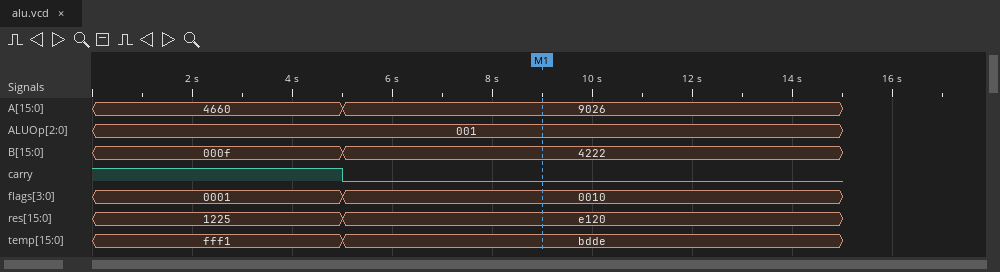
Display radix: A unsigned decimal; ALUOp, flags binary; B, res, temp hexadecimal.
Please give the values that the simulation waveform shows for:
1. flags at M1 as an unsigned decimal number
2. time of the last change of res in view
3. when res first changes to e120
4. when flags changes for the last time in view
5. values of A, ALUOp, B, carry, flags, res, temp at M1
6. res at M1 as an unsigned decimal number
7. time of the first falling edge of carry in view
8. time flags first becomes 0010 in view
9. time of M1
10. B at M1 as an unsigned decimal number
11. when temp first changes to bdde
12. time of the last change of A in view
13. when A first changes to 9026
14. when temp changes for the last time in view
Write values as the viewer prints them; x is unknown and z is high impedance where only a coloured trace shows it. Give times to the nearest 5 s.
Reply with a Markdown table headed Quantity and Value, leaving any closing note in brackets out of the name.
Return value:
| Quantity | Value |
|---|---|
| flags at M1 as an unsigned decimal number | 2 |
| time of the last change of res in view | 5 s |
| when res first changes to e120 | 5 s |
| when flags changes for the last time in view | 5 s |
| values of A, ALUOp, B, carry, flags, res, temp at M1 | A=9026, ALUOp=001, B=4222, carry=0, flags=0010, res=e120, temp=bdde |
| res at M1 as an unsigned decimal number | 57632 |
| time of the first falling edge of carry in view | 5 s |
| time flags first becomes 0010 in view | 5 s |
| time of M1 | 10 s |
| B at M1 as an unsigned decimal number | 16930 |
| when temp first changes to bdde | 5 s |
| time of the last change of A in view | 5 s |
| when A first changes to 9026 | 5 s |
| when temp changes for the last time in view | 5 s |
